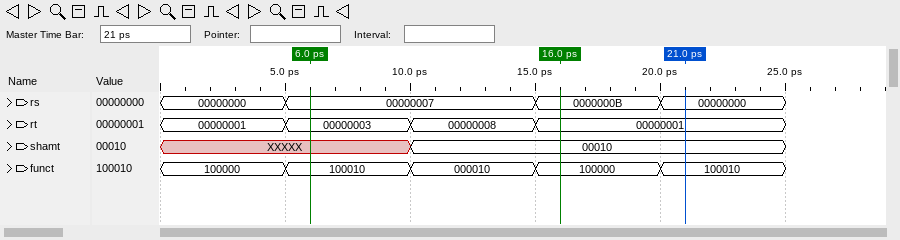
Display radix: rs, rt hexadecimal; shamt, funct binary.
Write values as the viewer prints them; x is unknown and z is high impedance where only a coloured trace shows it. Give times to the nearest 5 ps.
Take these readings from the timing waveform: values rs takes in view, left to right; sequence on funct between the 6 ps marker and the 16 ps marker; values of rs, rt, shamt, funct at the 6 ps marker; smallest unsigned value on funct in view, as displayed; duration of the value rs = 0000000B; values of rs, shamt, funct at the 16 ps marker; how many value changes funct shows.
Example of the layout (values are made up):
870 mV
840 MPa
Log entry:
00000000, 00000007, 0000000B, 00000000
100010, 000010, 100000
rs=00000007, rt=00000003, shamt=XXXXX, funct=100010
000010
5 ps
rs=0000000B, shamt=00010, funct=100000
4
